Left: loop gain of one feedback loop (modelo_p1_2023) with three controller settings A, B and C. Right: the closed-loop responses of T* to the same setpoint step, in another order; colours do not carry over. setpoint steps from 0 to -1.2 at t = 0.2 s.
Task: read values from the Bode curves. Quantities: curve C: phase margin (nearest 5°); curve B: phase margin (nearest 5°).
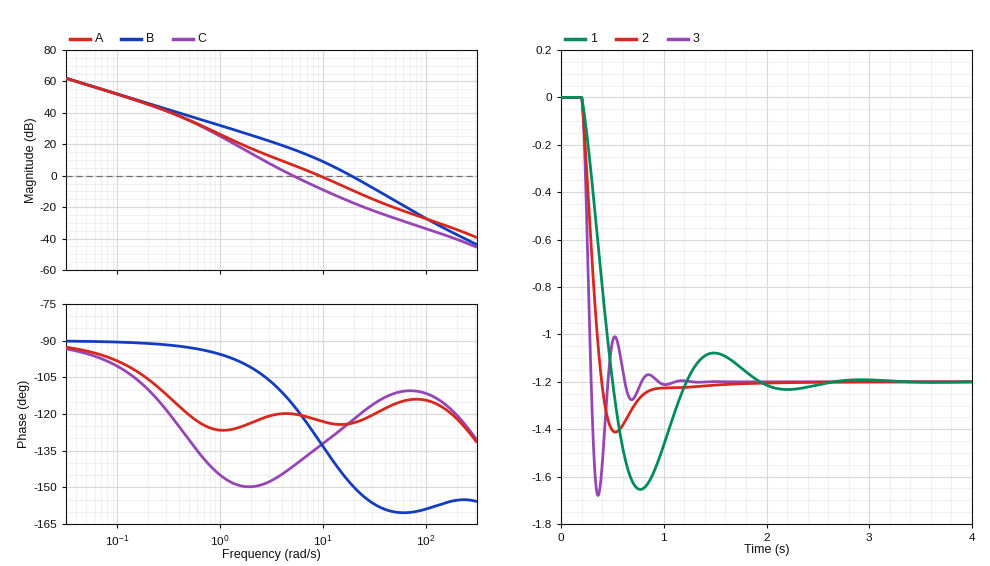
40°
30°
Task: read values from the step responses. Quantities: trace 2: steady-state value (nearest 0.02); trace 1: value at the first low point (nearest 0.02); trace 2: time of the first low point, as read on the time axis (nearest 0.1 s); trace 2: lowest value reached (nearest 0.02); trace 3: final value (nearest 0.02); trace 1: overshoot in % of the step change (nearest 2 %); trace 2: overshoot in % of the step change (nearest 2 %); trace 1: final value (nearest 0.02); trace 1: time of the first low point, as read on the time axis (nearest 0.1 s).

-1.20
-1.66
0.5 s
-1.42
-1.20
38 %
18 %
-1.20
0.8 s
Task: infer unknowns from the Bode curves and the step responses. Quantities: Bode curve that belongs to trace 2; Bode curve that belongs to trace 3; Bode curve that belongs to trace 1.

A
B
C
